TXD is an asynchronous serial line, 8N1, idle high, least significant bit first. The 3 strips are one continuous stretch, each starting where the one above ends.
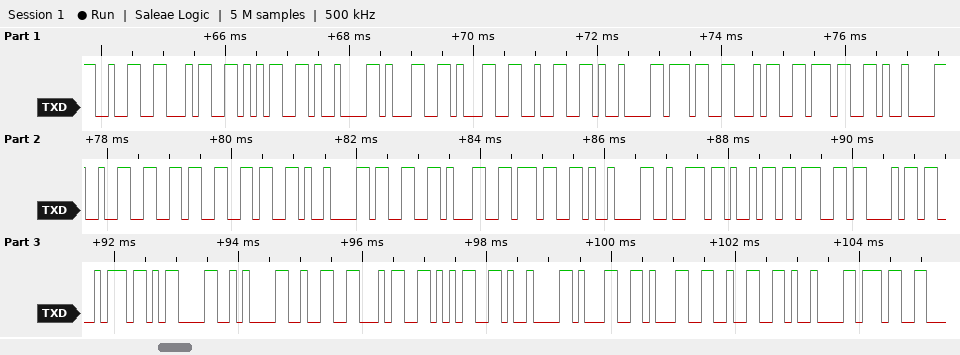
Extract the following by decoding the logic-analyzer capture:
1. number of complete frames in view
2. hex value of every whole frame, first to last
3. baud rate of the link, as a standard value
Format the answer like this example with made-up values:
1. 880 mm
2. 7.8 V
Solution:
1. 36
2. 0x32 0x34 0x35 0x09 0x31 0x31 0x32 0x09 0x37 0x34 0x37 0x09 0x32 0x36 0x36 0x09 0x33 0x31 0x37 0x09 0x72 0x69 0x67 0x68 0x74 0x0D 0x0A 0x32 0x34 0x35 0x09 0x31 0x31 0x32 0x09 0x37
3. 9600 baud
